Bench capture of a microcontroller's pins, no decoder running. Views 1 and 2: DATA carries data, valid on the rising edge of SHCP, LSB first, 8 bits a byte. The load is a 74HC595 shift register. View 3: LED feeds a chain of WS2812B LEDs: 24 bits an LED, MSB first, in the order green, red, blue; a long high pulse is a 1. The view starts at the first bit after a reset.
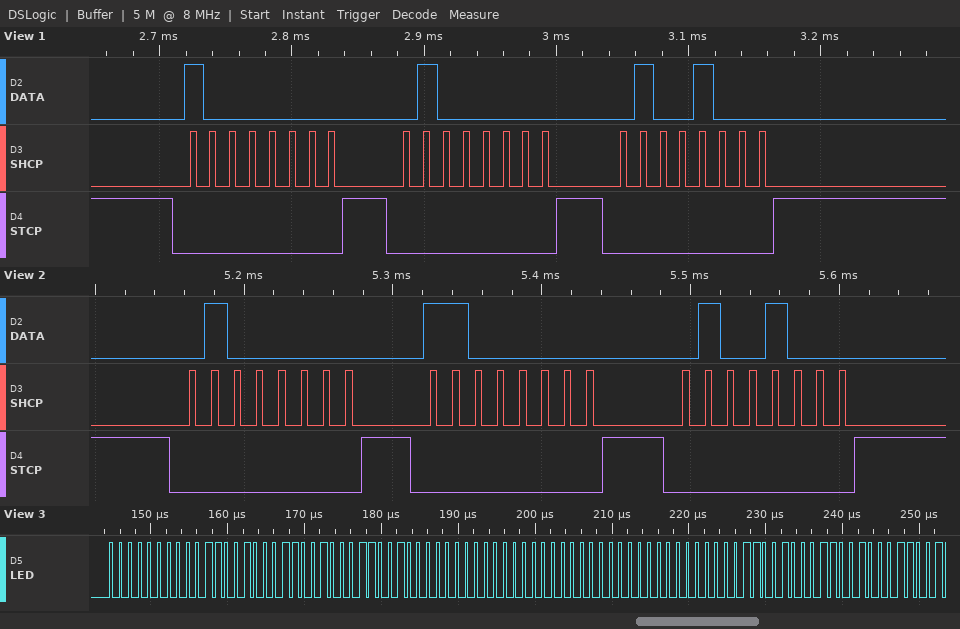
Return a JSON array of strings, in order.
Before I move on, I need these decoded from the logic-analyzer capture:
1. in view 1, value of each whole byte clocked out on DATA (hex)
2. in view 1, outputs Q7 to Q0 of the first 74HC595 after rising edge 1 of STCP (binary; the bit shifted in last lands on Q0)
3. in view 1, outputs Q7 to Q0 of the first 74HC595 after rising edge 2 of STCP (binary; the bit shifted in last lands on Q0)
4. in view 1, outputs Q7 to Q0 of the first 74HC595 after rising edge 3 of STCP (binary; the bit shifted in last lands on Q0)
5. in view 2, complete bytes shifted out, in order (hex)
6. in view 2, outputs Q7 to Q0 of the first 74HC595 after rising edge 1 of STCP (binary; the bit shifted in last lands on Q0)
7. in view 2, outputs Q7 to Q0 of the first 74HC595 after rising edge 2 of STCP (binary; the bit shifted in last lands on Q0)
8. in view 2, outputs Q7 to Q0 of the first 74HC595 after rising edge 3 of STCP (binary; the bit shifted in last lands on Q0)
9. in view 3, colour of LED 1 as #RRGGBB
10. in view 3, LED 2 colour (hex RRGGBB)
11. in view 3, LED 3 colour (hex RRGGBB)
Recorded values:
["01 02 12", "10000000", "01000000", "01001000", "02 03 12", "01000000", "11000000", "01001000", "#320032", "#003200", "#000032"]
